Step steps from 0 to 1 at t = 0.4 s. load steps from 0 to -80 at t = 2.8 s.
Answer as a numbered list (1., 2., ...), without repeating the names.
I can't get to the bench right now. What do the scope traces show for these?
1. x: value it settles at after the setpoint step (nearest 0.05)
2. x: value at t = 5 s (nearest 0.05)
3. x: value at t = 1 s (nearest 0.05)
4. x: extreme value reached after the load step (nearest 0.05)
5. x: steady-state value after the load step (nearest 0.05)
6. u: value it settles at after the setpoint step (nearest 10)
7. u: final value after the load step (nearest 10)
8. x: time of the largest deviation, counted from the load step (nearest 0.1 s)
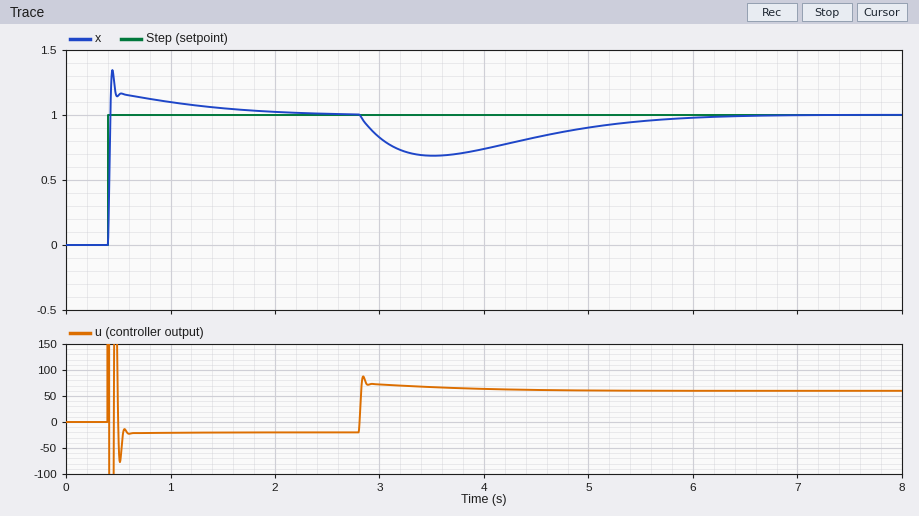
1. 1.00
2. 0.90
3. 1.10
4. 0.70
5. 1.00
6. -20
7. 60
8. 0.7 s
